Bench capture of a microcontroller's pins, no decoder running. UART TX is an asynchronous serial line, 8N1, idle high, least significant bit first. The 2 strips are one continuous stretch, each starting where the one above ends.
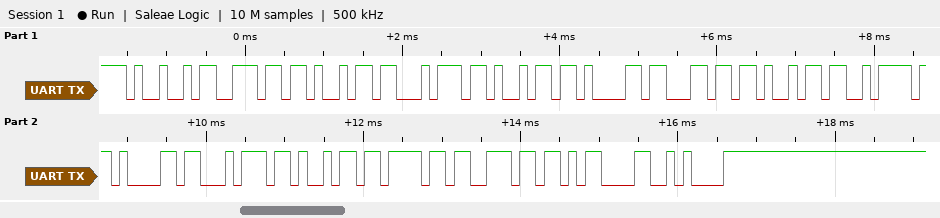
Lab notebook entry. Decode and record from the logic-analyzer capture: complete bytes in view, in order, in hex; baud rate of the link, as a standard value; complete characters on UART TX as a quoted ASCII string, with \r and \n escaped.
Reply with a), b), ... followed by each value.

a) 49 6E 69 74 69 61 6C 69 7A 61 74 69 6F 6E 0D 0A
b) 9600 baud
c) "Initialization\r\n"
